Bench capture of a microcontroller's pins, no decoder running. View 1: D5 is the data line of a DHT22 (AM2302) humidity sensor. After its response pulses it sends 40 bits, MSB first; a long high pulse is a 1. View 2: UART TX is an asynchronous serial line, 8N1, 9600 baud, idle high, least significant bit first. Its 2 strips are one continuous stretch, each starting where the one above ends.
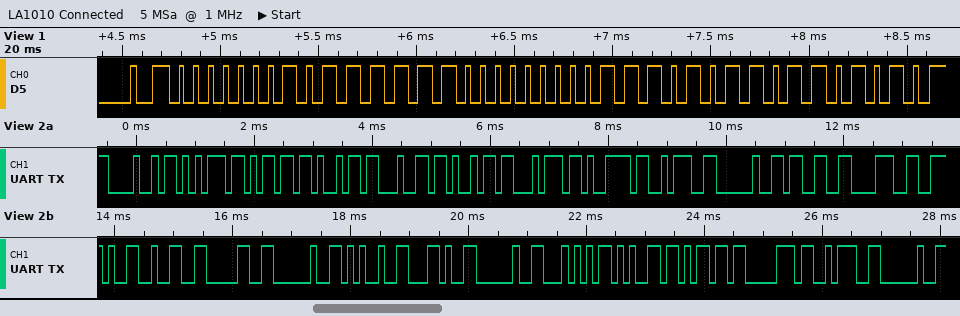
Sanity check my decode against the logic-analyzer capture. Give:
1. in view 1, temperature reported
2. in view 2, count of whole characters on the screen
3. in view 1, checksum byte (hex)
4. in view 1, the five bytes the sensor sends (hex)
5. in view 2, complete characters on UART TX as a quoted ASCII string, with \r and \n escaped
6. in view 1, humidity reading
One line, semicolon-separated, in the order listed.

23.5 °C; 25; 0x6A; 01 7E 00 EB 6A; "Humidity: 38.20 %, Temp: "; 38.2 %
